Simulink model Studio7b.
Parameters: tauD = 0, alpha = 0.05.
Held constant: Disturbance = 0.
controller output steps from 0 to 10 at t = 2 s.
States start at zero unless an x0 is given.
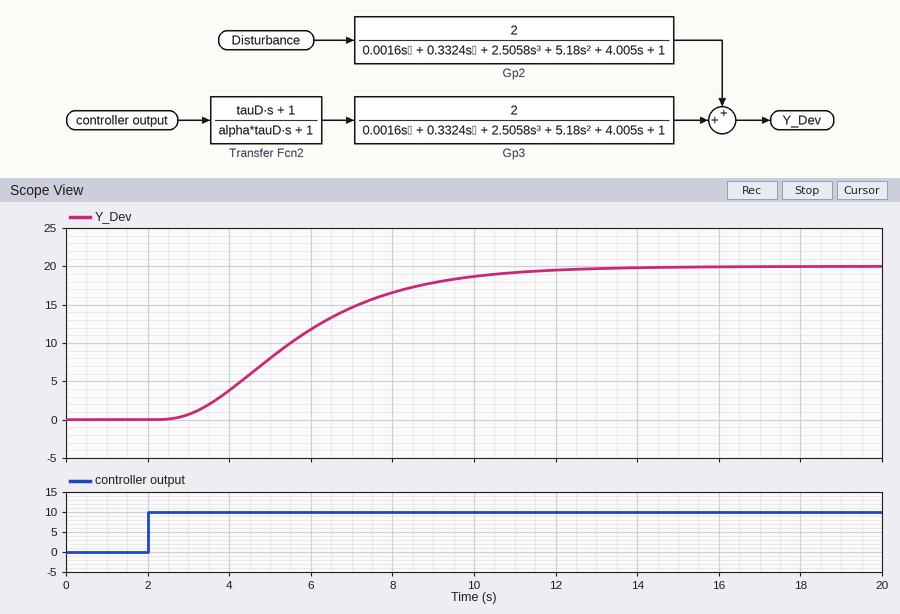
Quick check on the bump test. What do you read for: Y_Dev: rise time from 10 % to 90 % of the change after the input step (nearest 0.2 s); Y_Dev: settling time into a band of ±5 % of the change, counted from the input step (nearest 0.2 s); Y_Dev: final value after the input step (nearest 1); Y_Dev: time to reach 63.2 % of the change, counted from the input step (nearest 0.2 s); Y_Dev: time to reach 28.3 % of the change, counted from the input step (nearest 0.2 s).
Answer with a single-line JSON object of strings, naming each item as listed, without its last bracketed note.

{"Y_Dev: rise time from 10 % to 90 % of the change after the input step": "5.6 s", "Y_Dev: settling time into a band of ±5 % of the change, counted from the input step": "8.6 s", "Y_Dev: final value after the input step": "20", "Y_Dev: time to reach 63.2 % of the change, counted from the input step": "4.2 s", "Y_Dev: time to reach 28.3 % of the change, counted from the input step": "2.4 s"}
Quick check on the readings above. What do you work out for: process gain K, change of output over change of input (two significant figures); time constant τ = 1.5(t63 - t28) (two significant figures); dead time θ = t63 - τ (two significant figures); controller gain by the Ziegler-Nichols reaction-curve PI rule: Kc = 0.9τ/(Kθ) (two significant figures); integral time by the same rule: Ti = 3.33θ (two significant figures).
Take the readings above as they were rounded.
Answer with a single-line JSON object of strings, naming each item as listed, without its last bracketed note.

{"process gain K, change of output over change of input": "2.0", "time constant τ = 1.5(t63 - t28)": "2.7 s", "dead time θ = t63 - τ": "1.5 s", "controller gain by the Ziegler-Nichols reaction-curve PI rule: Kc = 0.9τ/(Kθ)": "0.81", "integral time by the same rule: Ti = 3.33θ": "5.0 s"}
